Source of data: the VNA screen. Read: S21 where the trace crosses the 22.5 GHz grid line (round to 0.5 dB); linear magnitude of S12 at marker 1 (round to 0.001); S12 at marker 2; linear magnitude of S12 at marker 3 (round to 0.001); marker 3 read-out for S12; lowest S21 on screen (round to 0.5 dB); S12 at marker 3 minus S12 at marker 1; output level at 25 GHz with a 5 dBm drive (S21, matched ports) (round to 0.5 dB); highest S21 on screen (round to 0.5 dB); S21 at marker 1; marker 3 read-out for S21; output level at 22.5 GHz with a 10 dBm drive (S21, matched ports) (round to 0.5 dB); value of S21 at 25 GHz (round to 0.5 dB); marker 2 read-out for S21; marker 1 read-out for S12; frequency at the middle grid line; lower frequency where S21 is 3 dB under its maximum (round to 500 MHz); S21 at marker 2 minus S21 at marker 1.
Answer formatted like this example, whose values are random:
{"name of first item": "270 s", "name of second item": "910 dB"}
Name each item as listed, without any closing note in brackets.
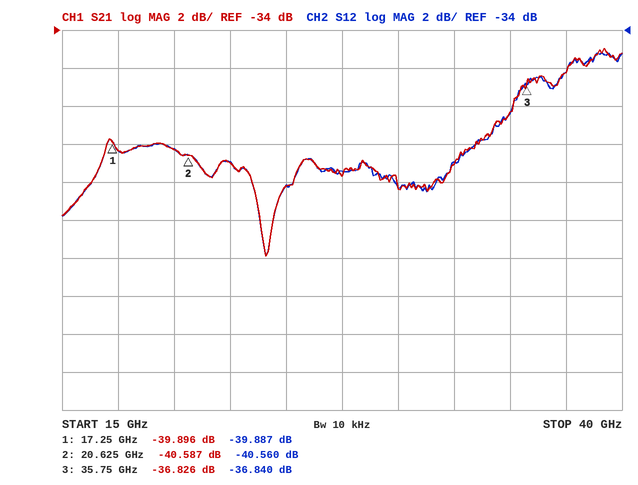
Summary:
{"S21 where the trace crosses the 22.5 GHz grid line": "-41.0 dB", "linear magnitude of S12 at marker 1": "0.010", "S12 at marker 2": "-40.560 dB", "linear magnitude of S12 at marker 3": "0.014", "marker 3 read-out for S12": "-36.840 dB", "lowest S21 on screen": "-46.0 dB", "S12 at marker 3 minus S12 at marker 1": "3.047 dB", "output level at 25 GHz with a 5 dBm drive (S21, matched ports)": "-37.0 dBm", "highest S21 on screen": "-35.0 dB", "S21 at marker 1": "-39.896 dB", "marker 3 read-out for S21": "-36.826 dB", "output level at 22.5 GHz with a 10 dBm drive (S21, matched ports)": "-31.0 dBm", "value of S21 at 25 GHz": "-42.0 dB", "marker 2 read-out for S21": "-40.587 dB", "marker 1 read-out for S12": "-39.887 dB", "frequency at the middle grid line": "27.5 GHz", "lower frequency where S21 is 3 dB under its maximum": "35.0 GHz", "S21 at marker 2 minus S21 at marker 1": "-0.691 dB"}
